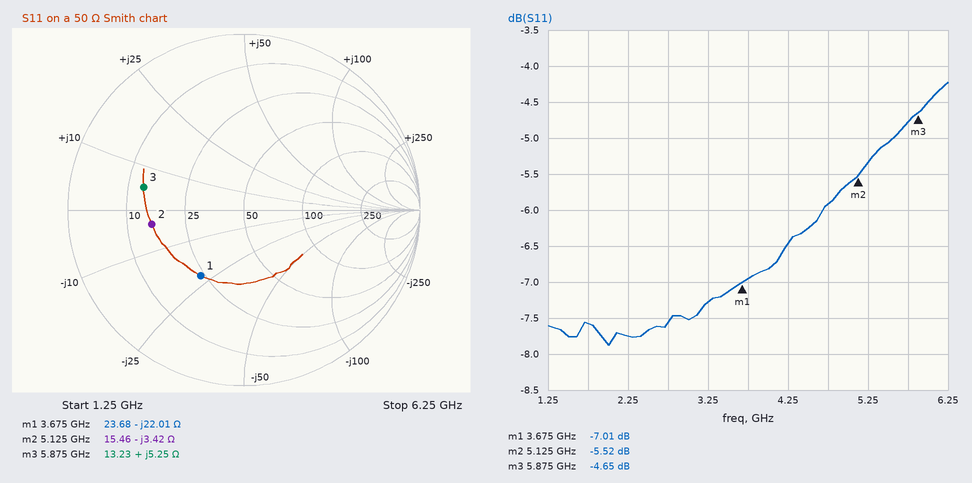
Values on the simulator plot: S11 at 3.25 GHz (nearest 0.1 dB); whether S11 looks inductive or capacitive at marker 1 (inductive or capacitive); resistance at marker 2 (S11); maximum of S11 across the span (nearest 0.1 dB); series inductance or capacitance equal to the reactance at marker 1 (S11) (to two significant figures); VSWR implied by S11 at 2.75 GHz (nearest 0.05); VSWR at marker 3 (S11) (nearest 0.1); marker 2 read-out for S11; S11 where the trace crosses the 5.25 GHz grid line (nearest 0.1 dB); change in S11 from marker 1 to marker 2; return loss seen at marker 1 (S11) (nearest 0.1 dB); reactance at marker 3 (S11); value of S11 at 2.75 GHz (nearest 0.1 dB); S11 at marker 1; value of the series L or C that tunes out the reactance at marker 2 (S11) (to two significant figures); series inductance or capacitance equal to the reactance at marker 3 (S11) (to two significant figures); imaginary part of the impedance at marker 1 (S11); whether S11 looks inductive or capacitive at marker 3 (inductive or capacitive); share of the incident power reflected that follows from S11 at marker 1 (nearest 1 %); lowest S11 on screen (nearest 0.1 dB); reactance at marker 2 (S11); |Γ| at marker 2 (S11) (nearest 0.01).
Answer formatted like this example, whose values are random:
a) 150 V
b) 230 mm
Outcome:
a) -7.3 dB
b) capacitive
c) 15.46 Ω
d) -4.2 dB
e) 2.0 pF
f) 2.45
g) 3.8
h) -5.52 dB
i) -5.3 dB
j) 1.49 dB
k) 7.0 dB
l) +5.25 Ω
m) -7.6 dB
n) -7.01 dB
o) 110 pH
p) 140 pH
q) -22.01 Ω
r) inductive
s) 20 %
t) -7.9 dB
u) -3.42 Ω
v) 0.53
